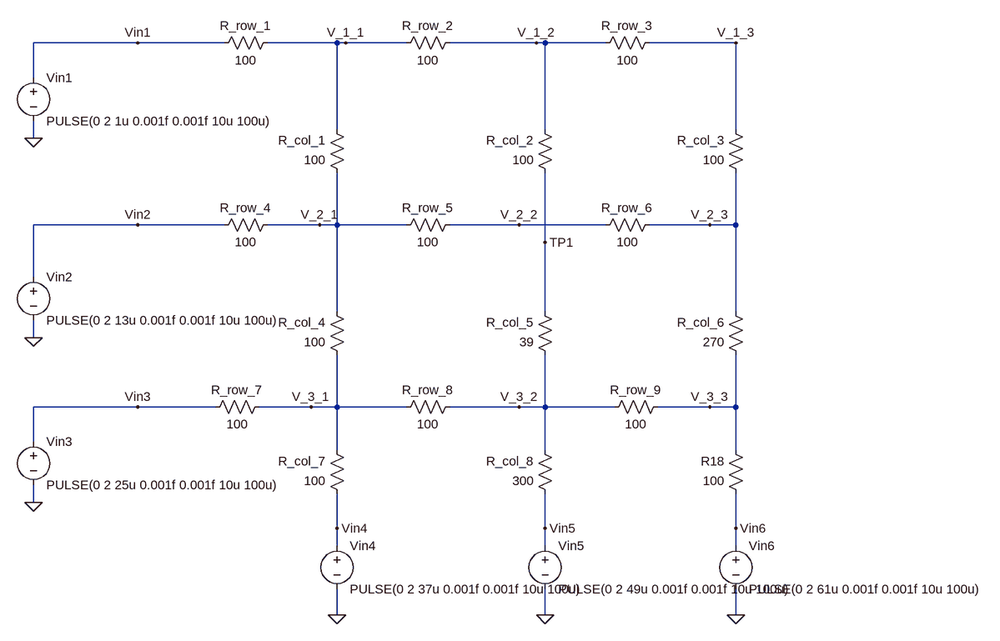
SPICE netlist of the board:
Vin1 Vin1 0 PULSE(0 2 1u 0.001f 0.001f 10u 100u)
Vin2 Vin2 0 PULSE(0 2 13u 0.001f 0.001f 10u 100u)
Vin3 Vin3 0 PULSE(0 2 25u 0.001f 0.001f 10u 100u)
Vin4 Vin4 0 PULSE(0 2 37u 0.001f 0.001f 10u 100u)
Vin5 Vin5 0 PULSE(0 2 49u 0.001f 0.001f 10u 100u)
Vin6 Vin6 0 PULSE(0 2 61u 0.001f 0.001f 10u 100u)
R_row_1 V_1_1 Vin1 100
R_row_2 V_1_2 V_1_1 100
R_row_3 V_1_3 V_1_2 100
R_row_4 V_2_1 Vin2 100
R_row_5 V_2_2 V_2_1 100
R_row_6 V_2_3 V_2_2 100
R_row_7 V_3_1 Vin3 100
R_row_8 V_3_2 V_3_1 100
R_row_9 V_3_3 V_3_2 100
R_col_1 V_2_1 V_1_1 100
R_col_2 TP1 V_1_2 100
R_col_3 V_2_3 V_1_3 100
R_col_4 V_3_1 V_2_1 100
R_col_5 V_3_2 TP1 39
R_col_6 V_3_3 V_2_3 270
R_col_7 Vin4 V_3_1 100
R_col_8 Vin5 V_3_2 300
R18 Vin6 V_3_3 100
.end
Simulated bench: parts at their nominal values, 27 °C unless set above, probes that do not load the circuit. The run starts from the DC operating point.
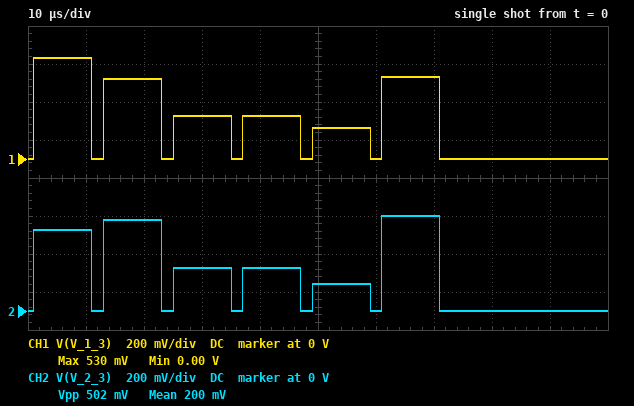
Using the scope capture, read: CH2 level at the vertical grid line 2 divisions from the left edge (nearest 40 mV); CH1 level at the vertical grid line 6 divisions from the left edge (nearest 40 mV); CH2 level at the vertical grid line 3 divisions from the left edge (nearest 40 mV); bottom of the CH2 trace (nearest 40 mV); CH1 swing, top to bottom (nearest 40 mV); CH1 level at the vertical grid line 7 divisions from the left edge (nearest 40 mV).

480 mV
0 V
240 mV
0 V
520 mV
440 mV
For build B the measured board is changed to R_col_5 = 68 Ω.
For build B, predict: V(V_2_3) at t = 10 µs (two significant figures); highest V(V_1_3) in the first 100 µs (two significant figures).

430 mV
550 mV
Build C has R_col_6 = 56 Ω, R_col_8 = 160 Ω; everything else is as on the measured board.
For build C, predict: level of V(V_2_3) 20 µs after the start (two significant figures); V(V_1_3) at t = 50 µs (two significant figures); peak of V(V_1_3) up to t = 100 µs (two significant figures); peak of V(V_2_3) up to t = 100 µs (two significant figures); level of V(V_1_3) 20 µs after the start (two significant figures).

330 mV
280 mV
570 mV
750 mV
320 mV
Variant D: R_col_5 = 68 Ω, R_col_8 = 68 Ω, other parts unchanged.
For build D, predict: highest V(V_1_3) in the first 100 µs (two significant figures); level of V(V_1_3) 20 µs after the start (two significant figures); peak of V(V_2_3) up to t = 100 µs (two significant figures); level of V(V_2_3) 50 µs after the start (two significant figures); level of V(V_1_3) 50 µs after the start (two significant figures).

510 mV
390 mV
450 mV
380 mV
430 mV
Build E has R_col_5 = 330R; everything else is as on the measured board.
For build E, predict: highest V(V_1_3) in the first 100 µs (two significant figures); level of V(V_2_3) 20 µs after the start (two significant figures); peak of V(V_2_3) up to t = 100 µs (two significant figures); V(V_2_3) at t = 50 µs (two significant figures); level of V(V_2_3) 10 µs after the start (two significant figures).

630 mV
500 mV
500 mV
120 mV
480 mV
